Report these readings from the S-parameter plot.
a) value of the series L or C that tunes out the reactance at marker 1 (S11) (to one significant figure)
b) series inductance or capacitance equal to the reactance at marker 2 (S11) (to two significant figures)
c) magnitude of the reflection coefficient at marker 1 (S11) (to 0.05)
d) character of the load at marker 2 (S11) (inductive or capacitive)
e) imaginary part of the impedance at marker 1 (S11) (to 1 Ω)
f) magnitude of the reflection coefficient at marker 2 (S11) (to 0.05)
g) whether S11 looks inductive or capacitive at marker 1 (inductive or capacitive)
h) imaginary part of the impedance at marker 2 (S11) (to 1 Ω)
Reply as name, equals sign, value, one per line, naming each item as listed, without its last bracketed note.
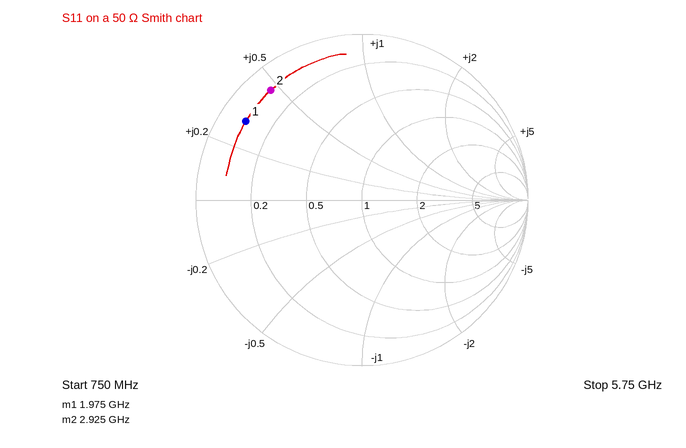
value of the series L or C that tunes out the reactance at marker 1 (S11) = 5 pF
series inductance or capacitance equal to the reactance at marker 2 (S11) = 1.3 nH
magnitude of the reflection coefficient at marker 1 (S11) = 0.85
character of the load at marker 2 (S11) = inductive
imaginary part of the impedance at marker 1 (S11) = +15 Ω
magnitude of the reflection coefficient at marker 2 (S11) = 0.85
whether S11 looks inductive or capacitive at marker 1 = inductive
imaginary part of the impedance at marker 2 (S11) = +23 Ω
